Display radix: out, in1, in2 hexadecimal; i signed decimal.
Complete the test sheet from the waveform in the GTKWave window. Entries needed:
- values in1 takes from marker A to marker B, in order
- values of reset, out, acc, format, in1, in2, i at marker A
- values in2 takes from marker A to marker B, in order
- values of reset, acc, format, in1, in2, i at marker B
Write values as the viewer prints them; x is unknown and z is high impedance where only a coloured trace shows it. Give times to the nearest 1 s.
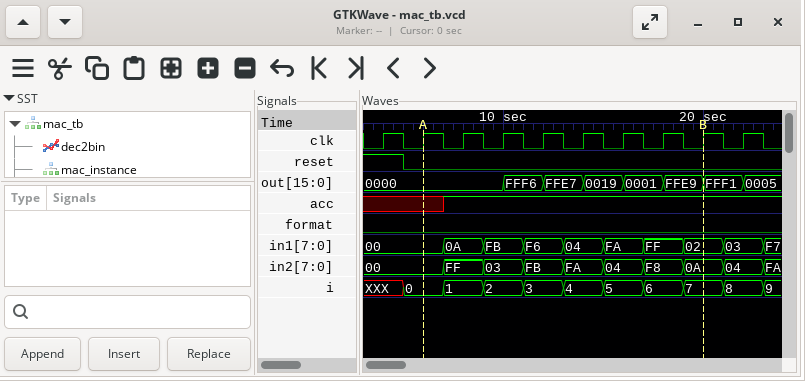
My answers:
00, 0A, FB, F6, 04, FA, FF, 02
reset=0, out=0000, acc=x, format=0, in1=00, in2=00, i=0
00, FF, 03, FB, FA, 04, F8, 0A
reset=0, acc=1, format=0, in1=02, in2=0A, i=7
